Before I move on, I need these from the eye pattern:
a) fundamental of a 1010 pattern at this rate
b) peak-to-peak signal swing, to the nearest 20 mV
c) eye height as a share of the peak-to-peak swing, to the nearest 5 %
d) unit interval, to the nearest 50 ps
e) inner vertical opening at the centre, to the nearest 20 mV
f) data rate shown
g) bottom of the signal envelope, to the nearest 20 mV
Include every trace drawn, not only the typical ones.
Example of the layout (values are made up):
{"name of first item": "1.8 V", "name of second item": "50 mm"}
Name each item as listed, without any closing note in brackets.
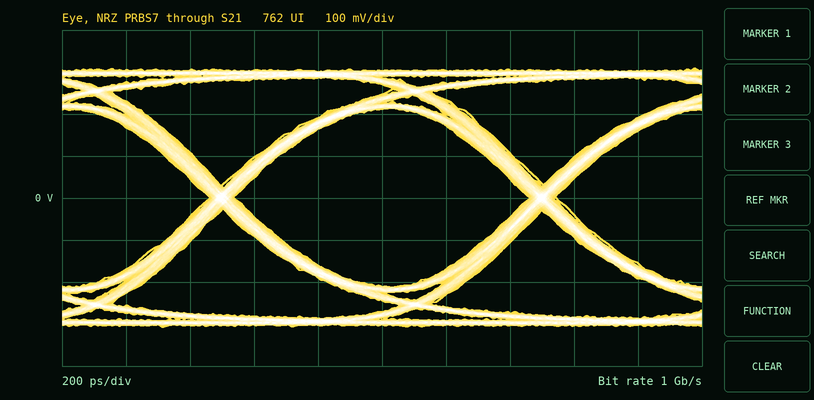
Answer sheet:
{"fundamental of a 1010 pattern at this rate": "500 MHz", "peak-to-peak signal swing, to the nearest 20 mV": "620 mV", "eye height as a share of the peak-to-peak swing, to the nearest 5 %": "70 %", "unit interval, to the nearest 50 ps": "1.00 ns", "inner vertical opening at the centre, to the nearest 20 mV": "420 mV", "data rate shown": "1 Gb/s", "bottom of the signal envelope, to the nearest 20 mV": "-300 mV"}
